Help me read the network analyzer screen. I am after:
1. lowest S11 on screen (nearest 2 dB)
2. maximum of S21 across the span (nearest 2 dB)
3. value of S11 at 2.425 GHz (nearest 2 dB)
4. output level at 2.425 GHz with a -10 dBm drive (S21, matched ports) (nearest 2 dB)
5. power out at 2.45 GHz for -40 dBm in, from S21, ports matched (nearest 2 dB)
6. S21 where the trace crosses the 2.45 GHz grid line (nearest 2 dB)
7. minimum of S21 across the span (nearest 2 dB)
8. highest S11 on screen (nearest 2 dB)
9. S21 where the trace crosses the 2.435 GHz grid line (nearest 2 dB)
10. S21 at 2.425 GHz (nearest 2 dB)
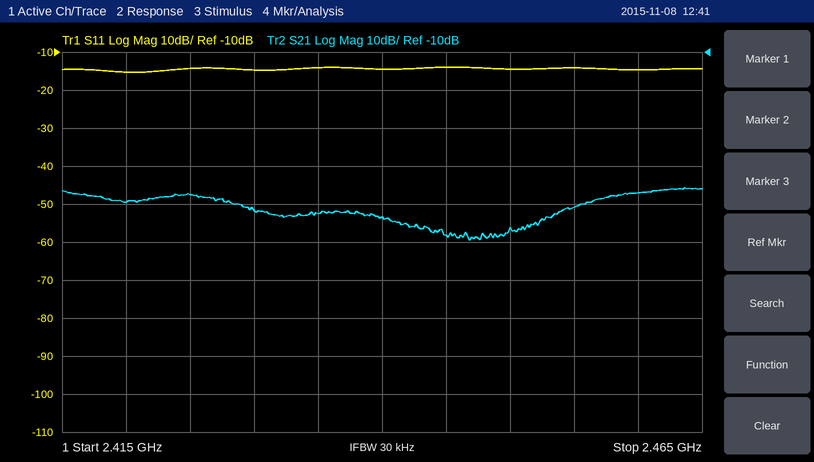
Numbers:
-16 dB
-46 dB
-14 dB
-58 dBm
-96 dBm
-56 dB
-60 dB
-14 dB
-52 dB
-48 dB
